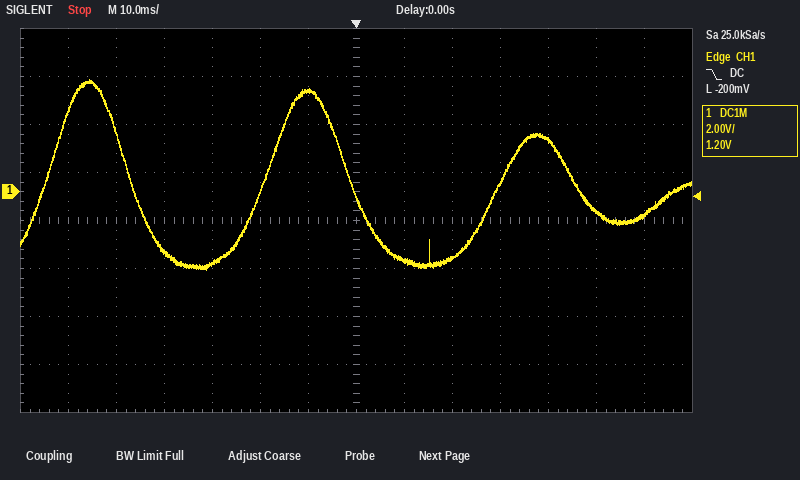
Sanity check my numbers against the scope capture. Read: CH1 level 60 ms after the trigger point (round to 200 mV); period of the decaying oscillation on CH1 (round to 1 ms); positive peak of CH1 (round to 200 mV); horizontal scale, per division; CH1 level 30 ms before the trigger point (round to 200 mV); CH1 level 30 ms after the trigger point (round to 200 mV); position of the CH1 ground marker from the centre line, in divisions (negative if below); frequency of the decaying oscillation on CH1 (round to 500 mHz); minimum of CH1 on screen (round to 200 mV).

-1.0 V
47 ms
4.6 V
10 ms
-3.0 V
400 mV
+0.6 div
21.5 Hz
-3.2 V
